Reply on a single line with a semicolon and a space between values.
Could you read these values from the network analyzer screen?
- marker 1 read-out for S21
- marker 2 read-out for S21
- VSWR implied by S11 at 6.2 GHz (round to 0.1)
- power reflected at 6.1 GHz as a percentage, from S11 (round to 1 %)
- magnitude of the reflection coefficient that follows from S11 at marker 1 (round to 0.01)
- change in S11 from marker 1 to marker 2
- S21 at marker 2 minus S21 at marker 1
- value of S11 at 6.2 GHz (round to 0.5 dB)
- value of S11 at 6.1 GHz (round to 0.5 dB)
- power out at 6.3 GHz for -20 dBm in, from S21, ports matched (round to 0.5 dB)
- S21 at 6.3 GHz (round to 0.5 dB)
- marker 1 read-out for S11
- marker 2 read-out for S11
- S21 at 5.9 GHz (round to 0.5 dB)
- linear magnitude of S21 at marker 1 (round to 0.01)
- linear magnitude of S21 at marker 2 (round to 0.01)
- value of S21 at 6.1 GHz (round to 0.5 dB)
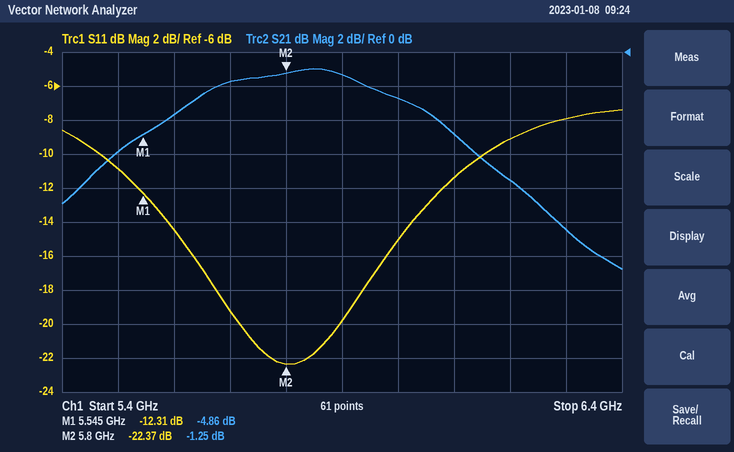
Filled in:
-4.86 dB; -1.25 dB; 2.1; 7 %; 0.24; -10.06 dB; 3.61 dB; -9.0 dB; -11.5 dB; -30.5 dBm; -10.5 dB; -12.31 dB; -22.37 dB; -1.5 dB; 0.57; 0.87; -5.0 dB
